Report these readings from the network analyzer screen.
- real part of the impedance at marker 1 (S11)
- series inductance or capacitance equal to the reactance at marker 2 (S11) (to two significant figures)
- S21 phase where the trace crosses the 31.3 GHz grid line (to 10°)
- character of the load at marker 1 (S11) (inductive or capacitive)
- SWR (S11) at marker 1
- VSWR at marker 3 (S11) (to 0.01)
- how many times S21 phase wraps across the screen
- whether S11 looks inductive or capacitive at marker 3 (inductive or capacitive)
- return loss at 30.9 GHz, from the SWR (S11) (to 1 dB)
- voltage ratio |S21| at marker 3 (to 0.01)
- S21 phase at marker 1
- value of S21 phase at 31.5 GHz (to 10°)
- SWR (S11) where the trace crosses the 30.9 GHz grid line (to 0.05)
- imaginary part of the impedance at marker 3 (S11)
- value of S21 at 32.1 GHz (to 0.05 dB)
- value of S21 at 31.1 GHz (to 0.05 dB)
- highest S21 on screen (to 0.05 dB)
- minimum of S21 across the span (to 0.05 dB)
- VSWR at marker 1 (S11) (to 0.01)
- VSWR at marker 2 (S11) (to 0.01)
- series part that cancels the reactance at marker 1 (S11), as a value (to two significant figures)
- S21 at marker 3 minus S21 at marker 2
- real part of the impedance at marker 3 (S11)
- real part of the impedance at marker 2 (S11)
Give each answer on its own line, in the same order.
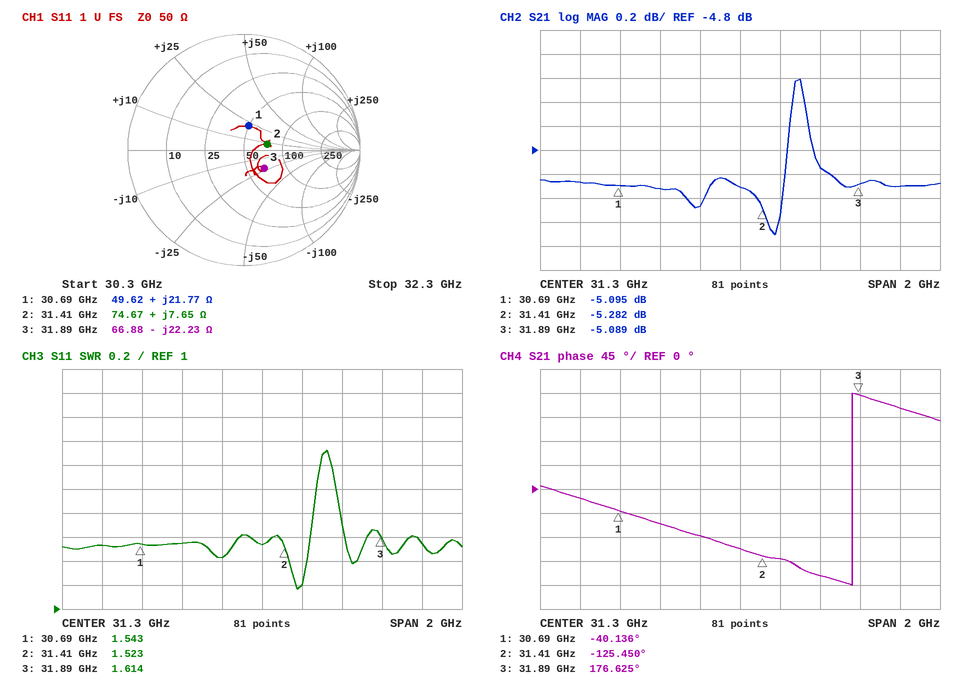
49.62 Ω
39 pH
-110°
inductive
1.543
1.61
1
capacitive
13 dB
0.56
-40.136°
-130°
1.55
-22.23 Ω
-5.10 dB
-5.25 dB
-4.20 dB
-5.50 dB
1.54
1.52
240 fF
0.193 dB
66.88 Ω
74.67 Ω
